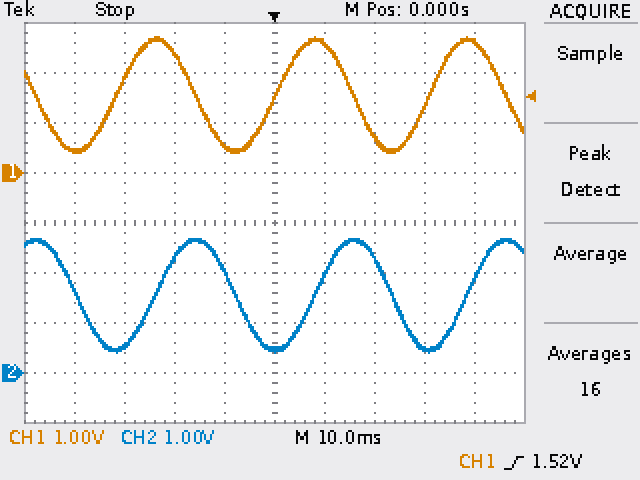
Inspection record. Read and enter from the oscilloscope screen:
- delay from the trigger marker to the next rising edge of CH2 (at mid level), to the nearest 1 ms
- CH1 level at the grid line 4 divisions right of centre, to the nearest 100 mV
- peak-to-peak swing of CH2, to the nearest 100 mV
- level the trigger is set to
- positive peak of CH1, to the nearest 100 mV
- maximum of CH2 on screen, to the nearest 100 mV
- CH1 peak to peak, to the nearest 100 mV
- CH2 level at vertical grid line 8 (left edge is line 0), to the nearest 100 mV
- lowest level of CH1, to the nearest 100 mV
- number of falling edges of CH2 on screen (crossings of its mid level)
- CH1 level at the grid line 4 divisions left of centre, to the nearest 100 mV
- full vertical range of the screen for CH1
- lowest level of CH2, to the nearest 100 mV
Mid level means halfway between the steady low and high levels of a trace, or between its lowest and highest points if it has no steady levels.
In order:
8 ms
2.6 V
2.3 V
1.52 V
2.7 V
2.7 V
2.3 V
500 mV
400 mV
3
400 mV
8 V
400 mV
